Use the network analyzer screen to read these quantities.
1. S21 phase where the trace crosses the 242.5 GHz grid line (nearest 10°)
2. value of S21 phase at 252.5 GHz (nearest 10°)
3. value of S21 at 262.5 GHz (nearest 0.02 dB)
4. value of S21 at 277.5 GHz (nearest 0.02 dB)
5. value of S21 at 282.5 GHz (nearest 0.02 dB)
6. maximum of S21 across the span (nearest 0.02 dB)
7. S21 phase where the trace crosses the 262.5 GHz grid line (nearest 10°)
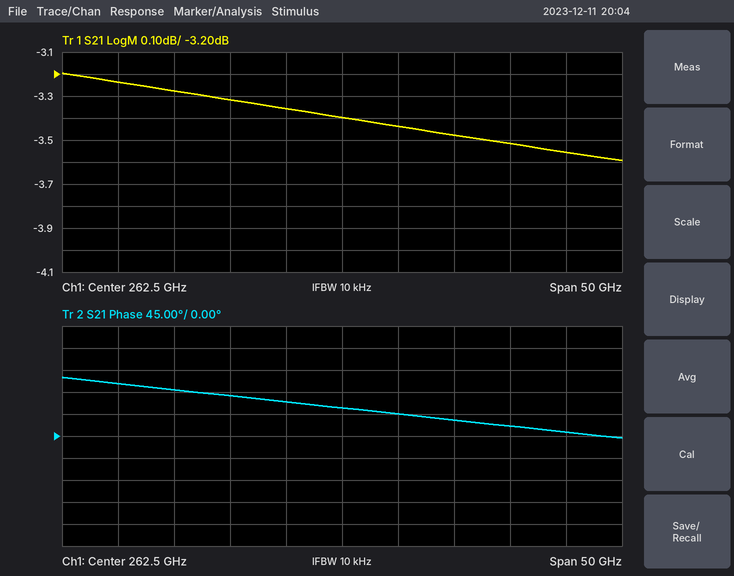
110°
80°
-3.40 dB
-3.52 dB
-3.56 dB
-3.20 dB
60°
